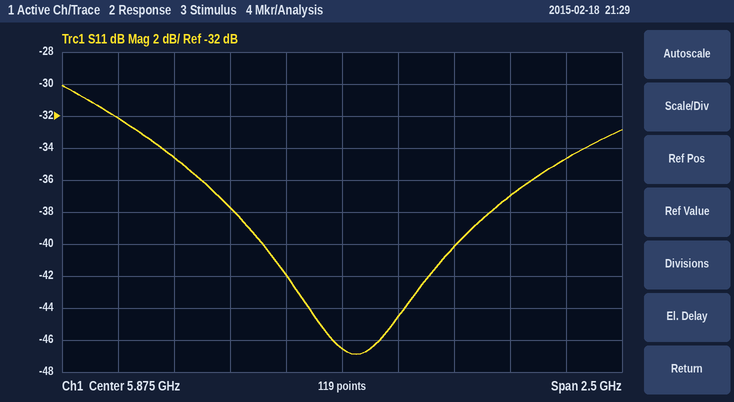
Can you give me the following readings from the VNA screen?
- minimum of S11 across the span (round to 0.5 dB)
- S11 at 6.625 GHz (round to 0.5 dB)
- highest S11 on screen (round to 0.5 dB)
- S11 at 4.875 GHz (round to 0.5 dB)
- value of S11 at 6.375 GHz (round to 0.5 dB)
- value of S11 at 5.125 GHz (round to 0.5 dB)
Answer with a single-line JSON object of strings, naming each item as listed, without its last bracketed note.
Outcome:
{"minimum of S11 across the span": "-47.0 dB", "S11 at 6.625 GHz": "-37.0 dB", "highest S11 on screen": "-30.0 dB", "S11 at 4.875 GHz": "-32.0 dB", "value of S11 at 6.375 GHz": "-40.0 dB", "value of S11 at 5.125 GHz": "-34.5 dB"}
